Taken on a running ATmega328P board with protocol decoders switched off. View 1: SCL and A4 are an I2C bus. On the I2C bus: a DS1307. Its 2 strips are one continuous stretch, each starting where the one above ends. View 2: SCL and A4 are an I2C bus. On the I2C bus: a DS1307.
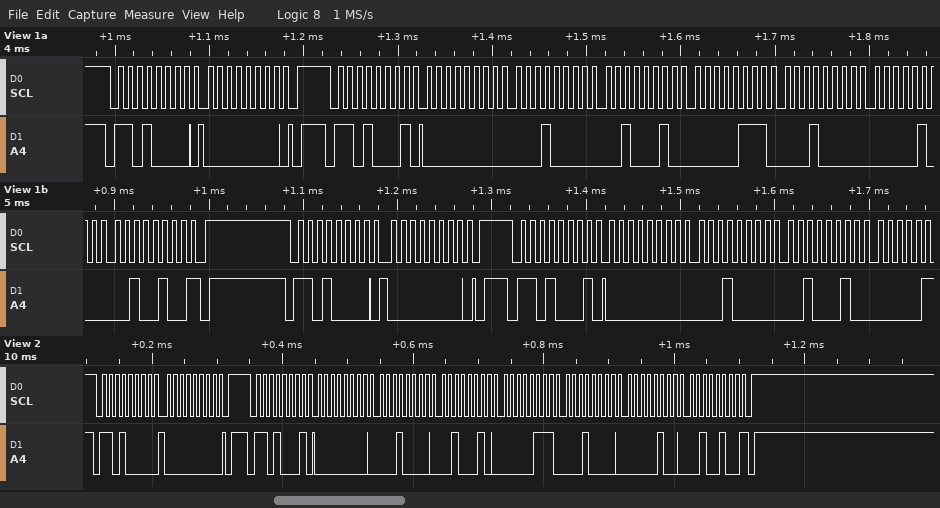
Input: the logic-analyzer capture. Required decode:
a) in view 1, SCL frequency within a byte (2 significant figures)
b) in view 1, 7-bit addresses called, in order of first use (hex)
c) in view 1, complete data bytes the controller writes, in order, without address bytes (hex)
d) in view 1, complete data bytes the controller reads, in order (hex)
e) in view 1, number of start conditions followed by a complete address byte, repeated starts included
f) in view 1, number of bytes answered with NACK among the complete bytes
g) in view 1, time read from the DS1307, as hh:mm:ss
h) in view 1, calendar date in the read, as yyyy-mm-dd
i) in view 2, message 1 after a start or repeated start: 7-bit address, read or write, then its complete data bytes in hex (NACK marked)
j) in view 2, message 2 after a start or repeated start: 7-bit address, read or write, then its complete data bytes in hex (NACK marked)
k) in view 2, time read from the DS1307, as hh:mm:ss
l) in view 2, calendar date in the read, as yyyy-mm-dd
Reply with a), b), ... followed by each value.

a) 100 kHz
b) 0x68
c) 00 00
d) 00 10 22 07 10 04 24 00 10 22
e) 4
f) 1
g) 22:10:00
h) 2024-04-10
i) 0x68 write: 00
j) 0x68 read: 00 10 22 07 10 04 24 NACK
k) 22:10:00
l) 2024-04-10
